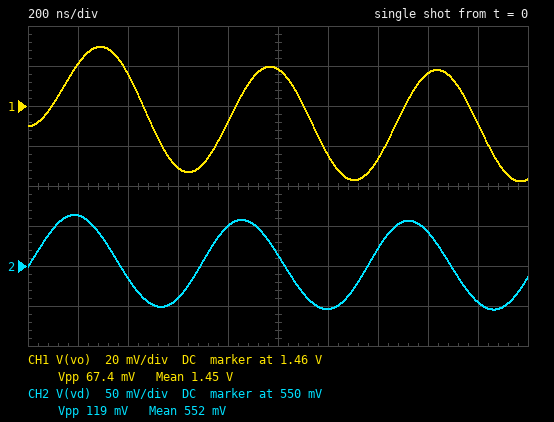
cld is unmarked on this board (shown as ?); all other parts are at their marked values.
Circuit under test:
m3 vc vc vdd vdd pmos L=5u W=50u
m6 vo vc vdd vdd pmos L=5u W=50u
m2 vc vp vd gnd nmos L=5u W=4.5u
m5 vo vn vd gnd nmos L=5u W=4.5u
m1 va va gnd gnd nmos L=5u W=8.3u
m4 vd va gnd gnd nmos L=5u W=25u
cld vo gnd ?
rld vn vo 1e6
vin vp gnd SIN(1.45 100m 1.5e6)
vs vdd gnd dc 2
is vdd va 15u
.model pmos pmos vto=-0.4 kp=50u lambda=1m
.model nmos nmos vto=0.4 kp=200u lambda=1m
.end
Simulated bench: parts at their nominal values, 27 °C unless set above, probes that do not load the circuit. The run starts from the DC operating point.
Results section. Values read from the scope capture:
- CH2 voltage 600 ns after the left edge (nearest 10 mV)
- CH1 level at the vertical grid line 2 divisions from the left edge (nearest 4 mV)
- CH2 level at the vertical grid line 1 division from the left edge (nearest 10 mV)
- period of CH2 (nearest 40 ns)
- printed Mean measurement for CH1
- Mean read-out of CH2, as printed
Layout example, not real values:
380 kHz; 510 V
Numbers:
510 mV; 1.476 V; 610 mV; 680 ns; 1.45 V; 552 mV
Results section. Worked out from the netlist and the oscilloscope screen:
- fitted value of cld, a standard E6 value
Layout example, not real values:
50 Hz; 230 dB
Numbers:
33 pF
